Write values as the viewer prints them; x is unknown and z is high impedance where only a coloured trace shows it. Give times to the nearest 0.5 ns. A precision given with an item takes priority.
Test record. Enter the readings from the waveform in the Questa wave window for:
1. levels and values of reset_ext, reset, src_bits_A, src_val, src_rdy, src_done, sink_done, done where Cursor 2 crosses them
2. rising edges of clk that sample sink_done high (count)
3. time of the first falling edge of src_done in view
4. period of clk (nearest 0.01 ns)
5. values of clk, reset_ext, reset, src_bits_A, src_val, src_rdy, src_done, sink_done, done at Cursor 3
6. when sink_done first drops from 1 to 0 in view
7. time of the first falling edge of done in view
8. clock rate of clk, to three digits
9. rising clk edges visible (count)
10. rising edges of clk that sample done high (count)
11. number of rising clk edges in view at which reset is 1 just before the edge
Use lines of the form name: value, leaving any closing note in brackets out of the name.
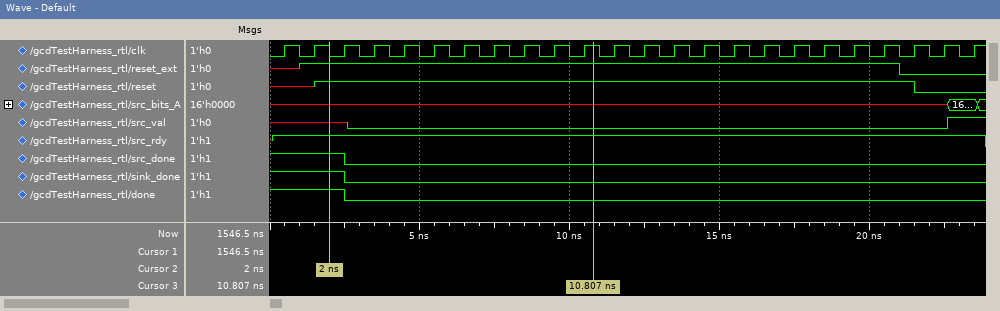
levels and values of reset_ext, reset, src_bits_A, src_val, src_rdy, src_done, sink_done, done where Cursor 2 crosses them: reset_ext=1, reset=1, src_bits_A=x, src_val=x, src_rdy=1, src_done=1, sink_done=1, done=1
rising edges of clk that sample sink_done high: 3
time of the first falling edge of src_done in view: 2.5 ns
period of clk: 1 ns
values of clk, reset_ext, reset, src_bits_A, src_val, src_rdy, src_done, sink_done, done at Cursor 3: clk=1, reset_ext=1, reset=1, src_bits_A=x, src_val=0, src_rdy=1, src_done=0, sink_done=0, done=0
when sink_done first drops from 1 to 0 in view: 2.5 ns
time of the first falling edge of done in view: 2.5 ns
clock rate of clk, to three digits: 1.00 GHz
rising clk edges visible: 24
rising edges of clk that sample done high: 3
number of rising clk edges in view at which reset is 1 just before the edge: 20
